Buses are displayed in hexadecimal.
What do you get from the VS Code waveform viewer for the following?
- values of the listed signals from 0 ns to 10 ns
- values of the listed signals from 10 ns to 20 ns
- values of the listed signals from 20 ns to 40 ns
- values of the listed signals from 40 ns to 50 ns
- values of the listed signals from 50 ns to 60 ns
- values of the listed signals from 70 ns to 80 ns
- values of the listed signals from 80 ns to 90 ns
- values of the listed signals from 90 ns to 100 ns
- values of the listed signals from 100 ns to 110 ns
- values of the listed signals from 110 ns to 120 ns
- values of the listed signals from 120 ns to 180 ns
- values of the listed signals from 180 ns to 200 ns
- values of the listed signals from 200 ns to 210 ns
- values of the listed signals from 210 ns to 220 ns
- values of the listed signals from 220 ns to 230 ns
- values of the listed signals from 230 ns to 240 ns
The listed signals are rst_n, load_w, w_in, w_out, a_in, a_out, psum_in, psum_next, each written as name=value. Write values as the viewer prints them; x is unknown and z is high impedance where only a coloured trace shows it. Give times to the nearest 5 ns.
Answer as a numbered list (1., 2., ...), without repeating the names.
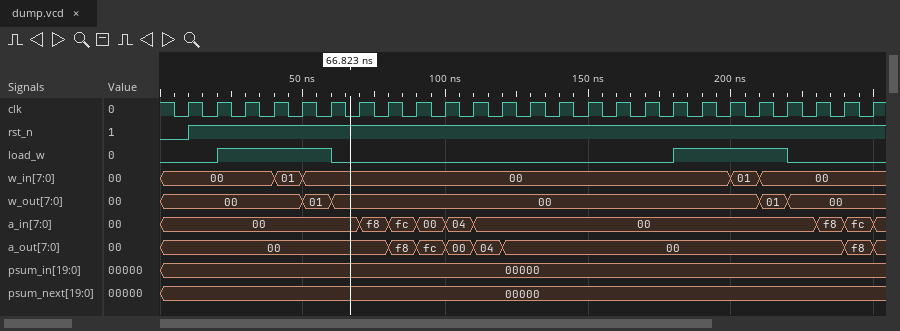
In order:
1. rst_n=0, load_w=0, w_in=00, w_out=00, a_in=00, a_out=00, psum_in=00000, psum_next=00000
2. rst_n=1, load_w=0, w_in=00, w_out=00, a_in=00, a_out=00, psum_in=00000, psum_next=00000
3. rst_n=1, load_w=1, w_in=00, w_out=00, a_in=00, a_out=00, psum_in=00000, psum_next=00000
4. rst_n=1, load_w=1, w_in=01, w_out=00, a_in=00, a_out=00, psum_in=00000, psum_next=00000
5. rst_n=1, load_w=1, w_in=00, w_out=01, a_in=00, a_out=00, psum_in=00000, psum_next=00000
6. rst_n=1, load_w=0, w_in=00, w_out=00, a_in=f8, a_out=00, psum_in=00000, psum_next=00000
7. rst_n=1, load_w=0, w_in=00, w_out=00, a_in=fc, a_out=f8, psum_in=00000, psum_next=00000
8. rst_n=1, load_w=0, w_in=00, w_out=00, a_in=00, a_out=fc, psum_in=00000, psum_next=00000
9. rst_n=1, load_w=0, w_in=00, w_out=00, a_in=04, a_out=00, psum_in=00000, psum_next=00000
10. rst_n=1, load_w=0, w_in=00, w_out=00, a_in=00, a_out=04, psum_in=00000, psum_next=00000
11. rst_n=1, load_w=0, w_in=00, w_out=00, a_in=00, a_out=00, psum_in=00000, psum_next=00000
12. rst_n=1, load_w=1, w_in=00, w_out=00, a_in=00, a_out=00, psum_in=00000, psum_next=00000
13. rst_n=1, load_w=1, w_in=01, w_out=00, a_in=00, a_out=00, psum_in=00000, psum_next=00000
14. rst_n=1, load_w=1, w_in=00, w_out=01, a_in=00, a_out=00, psum_in=00000, psum_next=00000
15. rst_n=1, load_w=0, w_in=00, w_out=00, a_in=00, a_out=00, psum_in=00000, psum_next=00000
16. rst_n=1, load_w=0, w_in=00, w_out=00, a_in=f8, a_out=00, psum_in=00000, psum_next=00000
